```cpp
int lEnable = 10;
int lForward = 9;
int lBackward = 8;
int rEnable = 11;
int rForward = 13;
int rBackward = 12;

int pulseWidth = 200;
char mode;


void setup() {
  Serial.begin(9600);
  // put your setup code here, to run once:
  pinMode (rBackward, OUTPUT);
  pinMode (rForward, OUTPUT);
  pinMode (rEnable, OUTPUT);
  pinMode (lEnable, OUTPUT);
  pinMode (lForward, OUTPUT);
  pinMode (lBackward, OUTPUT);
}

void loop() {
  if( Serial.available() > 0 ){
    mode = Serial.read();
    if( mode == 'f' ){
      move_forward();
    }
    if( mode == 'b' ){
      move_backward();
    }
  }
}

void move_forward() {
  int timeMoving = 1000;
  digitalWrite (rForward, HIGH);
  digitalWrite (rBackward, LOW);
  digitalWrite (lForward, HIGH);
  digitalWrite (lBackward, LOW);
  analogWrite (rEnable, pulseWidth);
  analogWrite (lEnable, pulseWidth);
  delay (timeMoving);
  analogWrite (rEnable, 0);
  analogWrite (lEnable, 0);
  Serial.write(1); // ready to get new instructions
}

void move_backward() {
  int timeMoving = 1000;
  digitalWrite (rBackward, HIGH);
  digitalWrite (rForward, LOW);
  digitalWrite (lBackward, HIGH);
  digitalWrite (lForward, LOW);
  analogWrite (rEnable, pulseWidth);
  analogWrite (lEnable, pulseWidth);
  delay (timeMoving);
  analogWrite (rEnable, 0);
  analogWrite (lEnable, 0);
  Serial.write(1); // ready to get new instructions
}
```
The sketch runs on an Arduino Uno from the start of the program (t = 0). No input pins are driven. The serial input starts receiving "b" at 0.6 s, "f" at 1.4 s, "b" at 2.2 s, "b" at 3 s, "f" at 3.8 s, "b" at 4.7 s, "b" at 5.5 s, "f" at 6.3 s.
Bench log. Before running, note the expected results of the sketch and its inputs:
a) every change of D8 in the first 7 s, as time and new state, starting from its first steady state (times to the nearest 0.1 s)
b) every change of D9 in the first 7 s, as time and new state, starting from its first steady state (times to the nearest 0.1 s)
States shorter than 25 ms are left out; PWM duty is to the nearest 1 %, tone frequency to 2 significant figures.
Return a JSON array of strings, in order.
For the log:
["0 s low; 0.6 s high; 1.6 s low; 2.6 s high; 4.6 s low; 5.6 s high", "0 s low; 1.6 s high; 2.6 s low; 4.6 s high; 5.6 s low"]
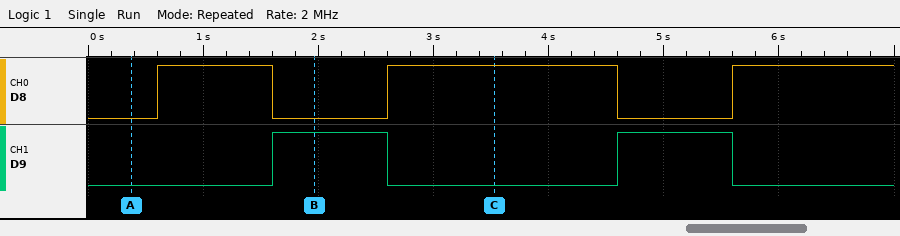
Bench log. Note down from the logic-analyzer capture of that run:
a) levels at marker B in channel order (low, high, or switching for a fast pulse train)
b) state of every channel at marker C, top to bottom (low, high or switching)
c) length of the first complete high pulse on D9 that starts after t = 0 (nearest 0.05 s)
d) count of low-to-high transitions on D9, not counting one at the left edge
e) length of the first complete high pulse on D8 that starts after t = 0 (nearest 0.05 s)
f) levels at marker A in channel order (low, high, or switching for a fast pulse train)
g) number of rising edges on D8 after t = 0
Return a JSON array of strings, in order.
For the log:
["D8 low, D9 high", "D8 high, D9 low", "1.00 s", "2", "1.00 s", "D8 low, D9 low", "3"]
